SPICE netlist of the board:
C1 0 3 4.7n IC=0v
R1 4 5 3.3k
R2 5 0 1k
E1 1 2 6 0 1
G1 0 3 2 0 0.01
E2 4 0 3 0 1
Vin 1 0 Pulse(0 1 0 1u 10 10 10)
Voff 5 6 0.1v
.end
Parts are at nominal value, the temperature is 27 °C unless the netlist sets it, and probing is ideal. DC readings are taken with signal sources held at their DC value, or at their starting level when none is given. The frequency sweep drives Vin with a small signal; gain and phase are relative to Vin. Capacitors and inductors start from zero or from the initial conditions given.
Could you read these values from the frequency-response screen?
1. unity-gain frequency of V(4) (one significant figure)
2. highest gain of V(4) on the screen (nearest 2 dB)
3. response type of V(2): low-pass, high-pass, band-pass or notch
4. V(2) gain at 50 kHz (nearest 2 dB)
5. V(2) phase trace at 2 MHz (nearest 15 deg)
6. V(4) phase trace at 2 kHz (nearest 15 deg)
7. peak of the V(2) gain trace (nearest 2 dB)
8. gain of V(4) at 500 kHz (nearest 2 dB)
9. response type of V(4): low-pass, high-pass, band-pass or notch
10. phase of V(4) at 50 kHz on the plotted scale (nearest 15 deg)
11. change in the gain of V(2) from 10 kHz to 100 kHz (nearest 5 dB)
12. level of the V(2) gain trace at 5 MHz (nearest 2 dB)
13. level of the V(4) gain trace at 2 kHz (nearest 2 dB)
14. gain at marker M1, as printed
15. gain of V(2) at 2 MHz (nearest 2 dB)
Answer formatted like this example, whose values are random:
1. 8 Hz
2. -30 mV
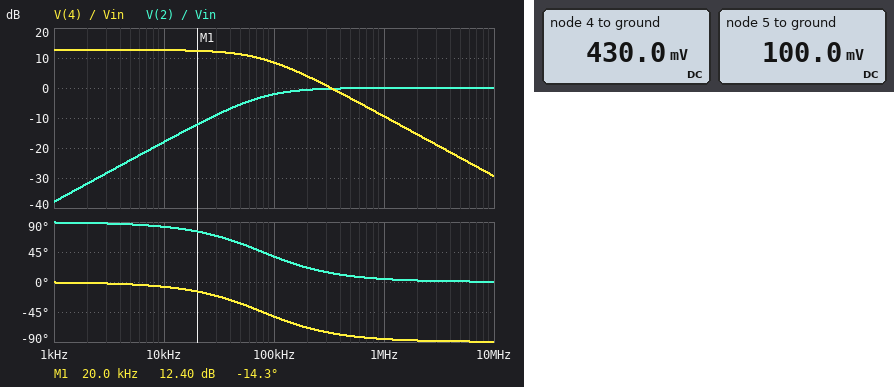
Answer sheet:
1. 300 kHz
2. 12 dB
3. high-pass
4. -6 dB
5. 0 deg
6. 0 deg
7. 0 dB
8. -4 dB
9. low-pass
10. -30 deg
11. 15 dB
12. 0 dB
13. 12 dB
14. 12.40 dB
15. 0 dB
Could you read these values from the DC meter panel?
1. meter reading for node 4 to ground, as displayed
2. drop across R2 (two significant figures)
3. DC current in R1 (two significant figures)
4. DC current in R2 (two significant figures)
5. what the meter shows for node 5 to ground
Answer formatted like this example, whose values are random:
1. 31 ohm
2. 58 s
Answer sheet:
1. 430.0 mV
2. 100 mV
3. 100 µA
4. 100 µA
5. 100.0 mV
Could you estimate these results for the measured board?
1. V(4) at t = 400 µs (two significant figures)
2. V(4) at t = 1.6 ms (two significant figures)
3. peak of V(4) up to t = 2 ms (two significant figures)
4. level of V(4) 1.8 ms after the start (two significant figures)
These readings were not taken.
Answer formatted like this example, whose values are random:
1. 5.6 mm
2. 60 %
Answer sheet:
1. 4.7 V
2. 4.7 V
3. 4.7 V
4. 4.7 V
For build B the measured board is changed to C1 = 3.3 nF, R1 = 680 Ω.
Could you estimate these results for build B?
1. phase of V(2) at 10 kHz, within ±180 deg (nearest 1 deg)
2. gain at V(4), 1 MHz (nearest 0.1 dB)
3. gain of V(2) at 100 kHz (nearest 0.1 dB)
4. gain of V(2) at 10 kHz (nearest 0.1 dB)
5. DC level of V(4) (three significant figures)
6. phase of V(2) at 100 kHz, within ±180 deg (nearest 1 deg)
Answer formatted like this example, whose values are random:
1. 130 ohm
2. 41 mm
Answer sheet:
1. 88 deg
2. -6.7 dB
3. -9.7 dB
4. -29.2 dB
5. 168 mV
6. 71 deg
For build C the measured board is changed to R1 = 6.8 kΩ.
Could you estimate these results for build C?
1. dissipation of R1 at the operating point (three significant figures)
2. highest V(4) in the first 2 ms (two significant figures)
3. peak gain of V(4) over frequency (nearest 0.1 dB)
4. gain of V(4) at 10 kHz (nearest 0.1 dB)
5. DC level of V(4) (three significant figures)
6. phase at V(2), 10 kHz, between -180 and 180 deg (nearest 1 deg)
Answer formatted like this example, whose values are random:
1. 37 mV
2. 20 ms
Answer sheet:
1. 68.0 µW
2. 8.6 V
3. 17.8 dB
4. 17.6 dB
5. 780 mV
6. 77 deg
